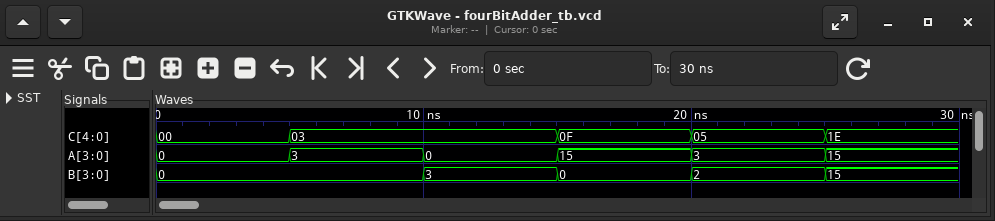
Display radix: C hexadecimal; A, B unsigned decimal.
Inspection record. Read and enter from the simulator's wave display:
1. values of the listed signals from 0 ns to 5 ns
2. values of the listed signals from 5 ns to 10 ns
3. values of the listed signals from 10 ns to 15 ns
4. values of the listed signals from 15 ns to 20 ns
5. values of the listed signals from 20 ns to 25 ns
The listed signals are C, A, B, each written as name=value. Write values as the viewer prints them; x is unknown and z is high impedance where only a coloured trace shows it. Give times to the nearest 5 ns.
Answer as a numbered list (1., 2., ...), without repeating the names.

1. C=00, A=0, B=0
2. C=03, A=3, B=0
3. C=03, A=0, B=3
4. C=0F, A=15, B=0
5. C=05, A=3, B=2
